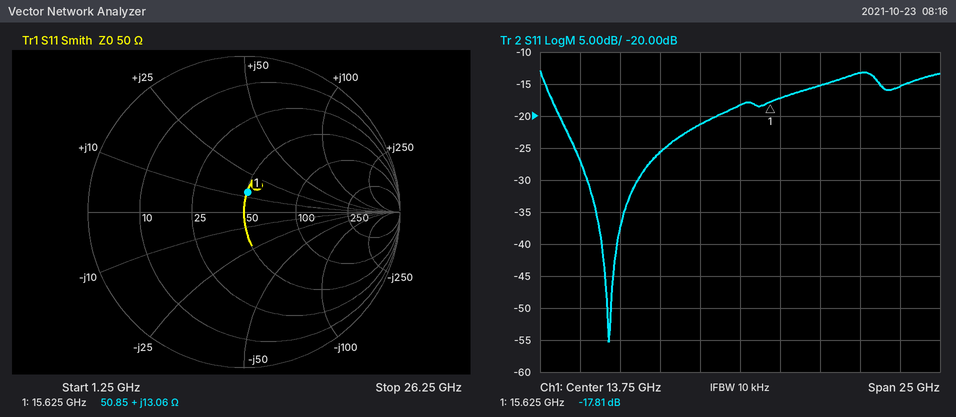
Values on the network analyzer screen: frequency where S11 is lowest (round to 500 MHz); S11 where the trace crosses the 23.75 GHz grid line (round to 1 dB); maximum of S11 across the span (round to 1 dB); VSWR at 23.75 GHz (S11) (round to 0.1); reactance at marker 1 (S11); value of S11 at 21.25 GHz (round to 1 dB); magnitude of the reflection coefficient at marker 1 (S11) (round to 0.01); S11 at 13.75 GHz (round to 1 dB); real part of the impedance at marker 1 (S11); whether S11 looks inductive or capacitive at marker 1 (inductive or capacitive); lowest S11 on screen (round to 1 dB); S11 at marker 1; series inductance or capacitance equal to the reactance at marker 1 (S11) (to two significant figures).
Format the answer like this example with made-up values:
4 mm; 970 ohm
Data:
5.5 GHz; -15 dB; -13 dB; 1.4; +13.06 Ω; -13 dB; 0.13; -18 dB; 50.85 Ω; inductive; -55 dB; -17.81 dB; 130 pH
